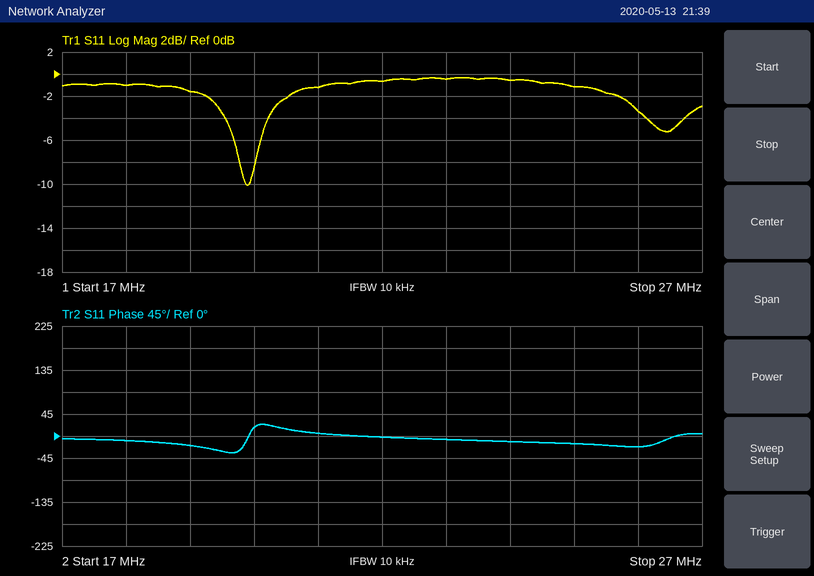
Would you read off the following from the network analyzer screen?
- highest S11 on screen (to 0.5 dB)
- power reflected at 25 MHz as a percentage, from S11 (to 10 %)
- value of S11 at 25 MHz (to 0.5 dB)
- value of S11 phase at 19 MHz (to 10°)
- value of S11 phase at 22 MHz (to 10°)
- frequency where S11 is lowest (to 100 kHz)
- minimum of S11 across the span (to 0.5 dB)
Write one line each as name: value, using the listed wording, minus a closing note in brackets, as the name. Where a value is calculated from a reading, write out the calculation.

highest S11 on screen: -0.5 dB
power reflected at 25 MHz as a percentage, from S11: 10^(-1/10) ≈ 79.4 %, so 80 % to the nearest 10 %
value of S11 at 25 MHz: -1.0 dB
value of S11 phase at 19 MHz: -20°
value of S11 phase at 22 MHz: 0°
frequency where S11 is lowest: 19.9 MHz
minimum of S11 across the span: -10.0 dB
